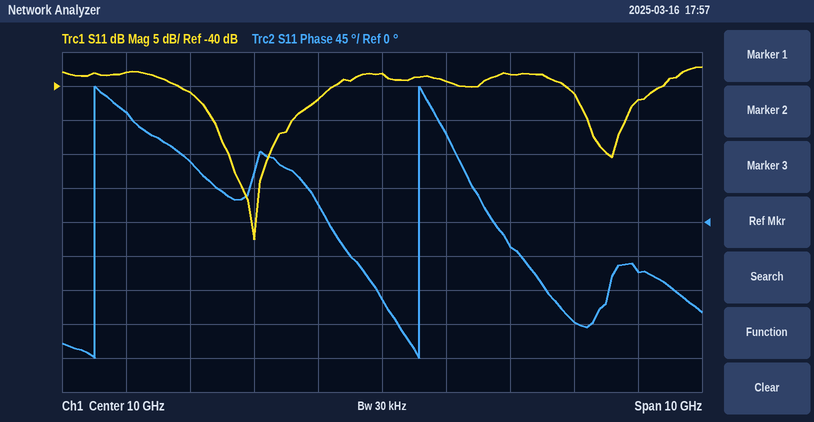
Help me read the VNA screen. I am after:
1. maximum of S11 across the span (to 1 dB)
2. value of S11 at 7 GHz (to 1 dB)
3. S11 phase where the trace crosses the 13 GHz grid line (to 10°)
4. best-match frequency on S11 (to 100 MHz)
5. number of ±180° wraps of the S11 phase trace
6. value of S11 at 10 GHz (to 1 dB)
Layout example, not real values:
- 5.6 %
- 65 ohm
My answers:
- -37 dB
- -41 dB
- -130°
- 8.0 GHz
- 2
- -38 dB
